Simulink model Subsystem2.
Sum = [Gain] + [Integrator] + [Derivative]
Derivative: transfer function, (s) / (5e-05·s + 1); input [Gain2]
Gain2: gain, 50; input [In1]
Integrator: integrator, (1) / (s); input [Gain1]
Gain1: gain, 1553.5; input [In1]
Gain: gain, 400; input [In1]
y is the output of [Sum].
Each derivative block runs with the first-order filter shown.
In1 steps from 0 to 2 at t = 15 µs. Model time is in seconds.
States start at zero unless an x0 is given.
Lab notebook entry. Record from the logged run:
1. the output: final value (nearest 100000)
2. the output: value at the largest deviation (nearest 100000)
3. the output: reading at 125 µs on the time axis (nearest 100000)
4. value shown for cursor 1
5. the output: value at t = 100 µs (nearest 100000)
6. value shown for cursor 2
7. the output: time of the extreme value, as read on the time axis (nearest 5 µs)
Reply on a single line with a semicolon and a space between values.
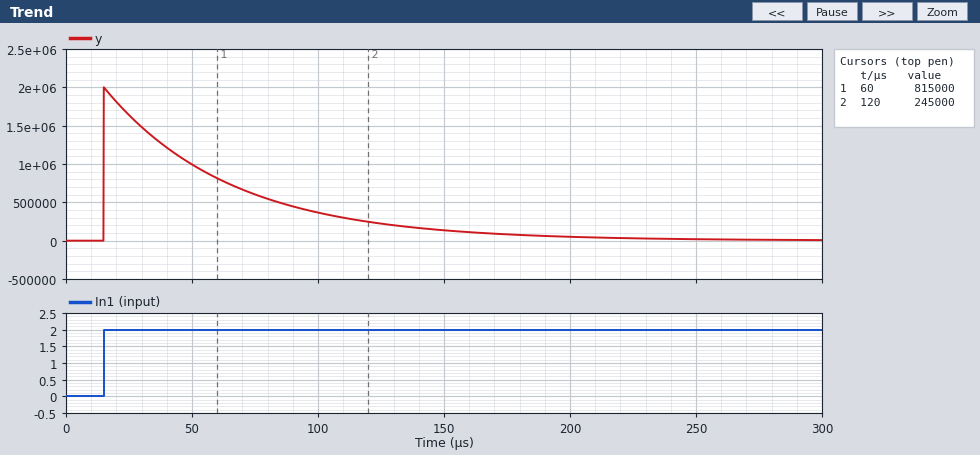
0; 2000000; 200000; 815000; 400000; 245000; 15 µs
